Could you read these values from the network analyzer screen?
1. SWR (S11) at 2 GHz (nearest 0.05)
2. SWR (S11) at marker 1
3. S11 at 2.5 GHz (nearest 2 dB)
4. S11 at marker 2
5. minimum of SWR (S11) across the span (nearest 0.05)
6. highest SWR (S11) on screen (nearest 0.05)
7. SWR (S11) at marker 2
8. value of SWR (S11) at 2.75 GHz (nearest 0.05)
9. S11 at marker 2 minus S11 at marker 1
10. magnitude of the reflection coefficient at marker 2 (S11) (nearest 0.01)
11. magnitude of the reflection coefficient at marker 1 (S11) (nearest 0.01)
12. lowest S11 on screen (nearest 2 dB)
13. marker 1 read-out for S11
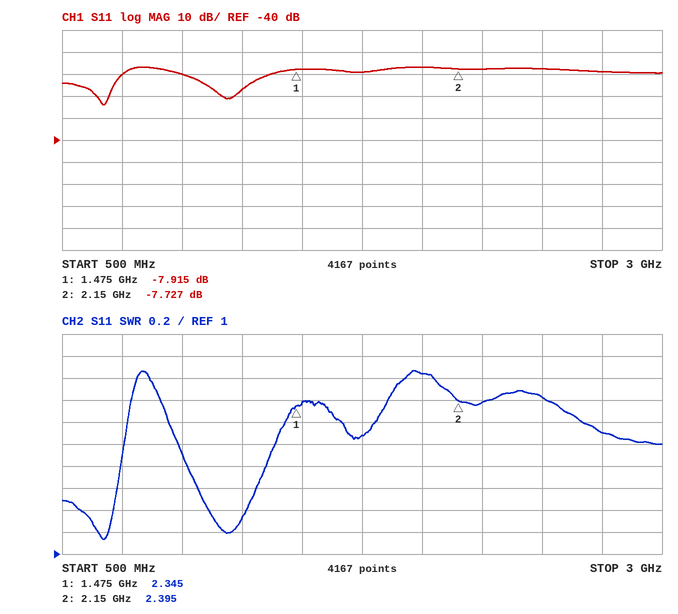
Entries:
2.65
2.345
-8 dB
-7.727 dB
1.15
2.65
2.395
2.10
0.188 dB
0.41
0.40
-24 dB
-7.915 dB
